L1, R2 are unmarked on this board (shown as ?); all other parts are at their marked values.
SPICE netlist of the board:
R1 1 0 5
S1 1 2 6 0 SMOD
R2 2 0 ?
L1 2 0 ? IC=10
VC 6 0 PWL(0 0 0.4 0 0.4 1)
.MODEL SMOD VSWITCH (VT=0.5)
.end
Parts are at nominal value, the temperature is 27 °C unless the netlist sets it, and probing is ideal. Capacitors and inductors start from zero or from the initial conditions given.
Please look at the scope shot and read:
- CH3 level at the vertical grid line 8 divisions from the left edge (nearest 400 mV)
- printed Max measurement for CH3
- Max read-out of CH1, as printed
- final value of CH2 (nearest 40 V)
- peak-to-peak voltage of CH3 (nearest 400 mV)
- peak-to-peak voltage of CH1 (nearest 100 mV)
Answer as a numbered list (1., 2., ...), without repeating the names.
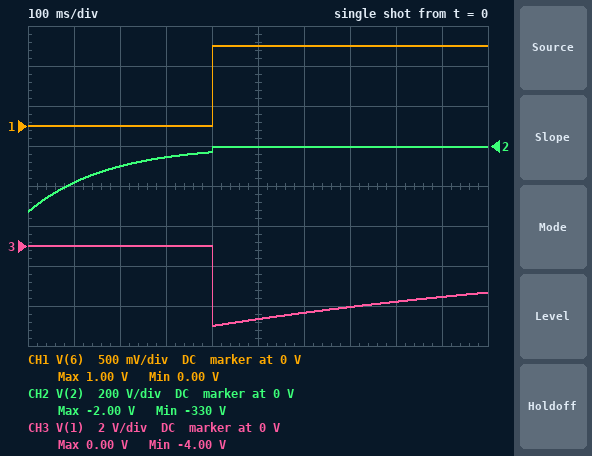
1. -2.8 V
2. 0.00 V
3. 1.00 V
4. 0 V
5. 4.0 V
6. 1.0 V
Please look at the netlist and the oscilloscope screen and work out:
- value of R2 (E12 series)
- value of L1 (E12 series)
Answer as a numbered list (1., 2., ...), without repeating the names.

1. 33 Ω
2. 5.6 H
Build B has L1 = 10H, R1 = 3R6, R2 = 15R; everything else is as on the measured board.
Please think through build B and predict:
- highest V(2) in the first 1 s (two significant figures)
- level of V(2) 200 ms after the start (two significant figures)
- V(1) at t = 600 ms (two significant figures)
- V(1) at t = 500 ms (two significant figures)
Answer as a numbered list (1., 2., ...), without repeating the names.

1. -16 V
2. -110 V
3. -14 V
4. -15 V
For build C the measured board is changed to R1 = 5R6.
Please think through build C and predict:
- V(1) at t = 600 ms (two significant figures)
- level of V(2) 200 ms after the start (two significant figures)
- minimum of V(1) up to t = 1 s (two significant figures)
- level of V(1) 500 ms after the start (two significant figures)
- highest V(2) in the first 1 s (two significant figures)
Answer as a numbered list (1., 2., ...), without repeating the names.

1. -3.6 V
2. -100 V
3. -4.4 V
4. -4.0 V
5. -2.9 V
